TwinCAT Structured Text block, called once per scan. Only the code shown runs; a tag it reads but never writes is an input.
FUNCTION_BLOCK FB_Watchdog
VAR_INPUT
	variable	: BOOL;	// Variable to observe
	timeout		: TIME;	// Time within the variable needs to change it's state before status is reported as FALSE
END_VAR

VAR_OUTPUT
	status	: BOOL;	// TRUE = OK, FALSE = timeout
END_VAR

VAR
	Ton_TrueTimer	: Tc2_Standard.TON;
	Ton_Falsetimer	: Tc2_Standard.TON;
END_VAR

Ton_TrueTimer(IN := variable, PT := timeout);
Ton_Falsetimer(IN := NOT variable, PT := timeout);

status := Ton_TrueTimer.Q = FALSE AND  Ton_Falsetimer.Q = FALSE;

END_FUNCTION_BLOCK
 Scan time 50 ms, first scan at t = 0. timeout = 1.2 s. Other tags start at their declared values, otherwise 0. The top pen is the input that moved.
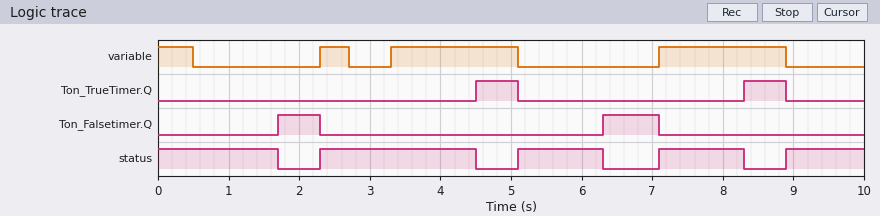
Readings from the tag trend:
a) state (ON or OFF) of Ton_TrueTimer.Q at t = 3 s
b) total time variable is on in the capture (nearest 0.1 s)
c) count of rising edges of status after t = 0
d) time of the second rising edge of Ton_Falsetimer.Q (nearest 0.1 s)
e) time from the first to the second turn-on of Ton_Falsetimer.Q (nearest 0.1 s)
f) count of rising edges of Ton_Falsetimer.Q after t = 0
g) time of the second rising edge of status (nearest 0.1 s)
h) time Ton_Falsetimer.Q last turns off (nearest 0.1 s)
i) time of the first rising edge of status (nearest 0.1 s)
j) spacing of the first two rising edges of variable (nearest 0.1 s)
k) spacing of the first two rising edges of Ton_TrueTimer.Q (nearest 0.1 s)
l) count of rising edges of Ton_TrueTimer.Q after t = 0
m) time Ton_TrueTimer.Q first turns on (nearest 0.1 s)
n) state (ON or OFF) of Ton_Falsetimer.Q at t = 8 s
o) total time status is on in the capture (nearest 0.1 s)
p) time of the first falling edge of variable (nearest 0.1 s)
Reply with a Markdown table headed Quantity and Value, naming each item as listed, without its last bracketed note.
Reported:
| Quantity | Value |
|---|---|
| state (ON or OFF) of Ton_TrueTimer.Q at t = 3 s | OFF |
| total time variable is on in the capture | 4.5 s |
| count of rising edges of status after t = 0 | 4 |
| time of the second rising edge of Ton_Falsetimer.Q | 6.3 s |
| time from the first to the second turn-on of Ton_Falsetimer.Q | 4.6 s |
| count of rising edges of Ton_Falsetimer.Q after t = 0 | 2 |
| time of the second rising edge of status | 5.1 s |
| time Ton_Falsetimer.Q last turns off | 7.1 s |
| time of the first rising edge of status | 2.3 s |
| spacing of the first two rising edges of variable | 1.0 s |
| spacing of the first two rising edges of Ton_TrueTimer.Q | 3.8 s |
| count of rising edges of Ton_TrueTimer.Q after t = 0 | 2 |
| time Ton_TrueTimer.Q first turns on | 4.5 s |
| state (ON or OFF) of Ton_Falsetimer.Q at t = 8 s | OFF |
| total time status is on in the capture | 7.4 s |
| time of the first falling edge of variable | 0.5 s |
